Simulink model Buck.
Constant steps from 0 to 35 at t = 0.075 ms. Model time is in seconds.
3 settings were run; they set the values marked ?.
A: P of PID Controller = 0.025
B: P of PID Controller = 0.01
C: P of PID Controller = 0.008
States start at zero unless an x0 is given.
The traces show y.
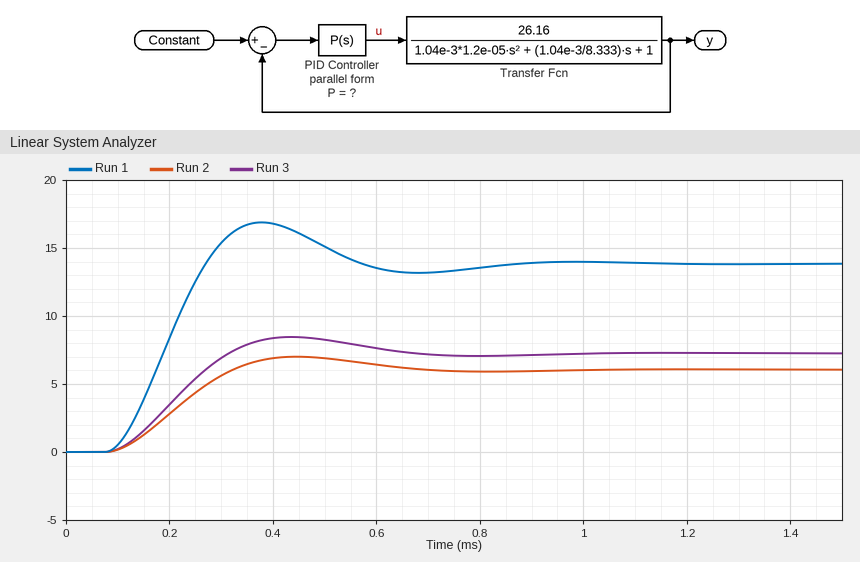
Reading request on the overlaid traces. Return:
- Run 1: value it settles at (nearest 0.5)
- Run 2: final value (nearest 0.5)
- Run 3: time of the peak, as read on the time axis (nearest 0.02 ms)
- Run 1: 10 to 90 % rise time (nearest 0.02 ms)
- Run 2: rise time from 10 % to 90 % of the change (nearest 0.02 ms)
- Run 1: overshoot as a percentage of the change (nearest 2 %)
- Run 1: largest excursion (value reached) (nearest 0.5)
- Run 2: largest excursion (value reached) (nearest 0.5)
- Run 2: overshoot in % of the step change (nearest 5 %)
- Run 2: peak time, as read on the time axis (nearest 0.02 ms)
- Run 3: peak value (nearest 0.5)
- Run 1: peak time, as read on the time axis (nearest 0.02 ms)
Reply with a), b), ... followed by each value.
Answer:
a) 14.0
b) 6.0
c) 0.44 ms
d) 0.14 ms
e) 0.16 ms
f) 22 %
g) 17.0
h) 7.0
i) 15 %
j) 0.44 ms
k) 8.5
l) 0.38 ms
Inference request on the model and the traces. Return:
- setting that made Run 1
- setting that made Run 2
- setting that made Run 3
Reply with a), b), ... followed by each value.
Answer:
a) A
b) C
c) B
